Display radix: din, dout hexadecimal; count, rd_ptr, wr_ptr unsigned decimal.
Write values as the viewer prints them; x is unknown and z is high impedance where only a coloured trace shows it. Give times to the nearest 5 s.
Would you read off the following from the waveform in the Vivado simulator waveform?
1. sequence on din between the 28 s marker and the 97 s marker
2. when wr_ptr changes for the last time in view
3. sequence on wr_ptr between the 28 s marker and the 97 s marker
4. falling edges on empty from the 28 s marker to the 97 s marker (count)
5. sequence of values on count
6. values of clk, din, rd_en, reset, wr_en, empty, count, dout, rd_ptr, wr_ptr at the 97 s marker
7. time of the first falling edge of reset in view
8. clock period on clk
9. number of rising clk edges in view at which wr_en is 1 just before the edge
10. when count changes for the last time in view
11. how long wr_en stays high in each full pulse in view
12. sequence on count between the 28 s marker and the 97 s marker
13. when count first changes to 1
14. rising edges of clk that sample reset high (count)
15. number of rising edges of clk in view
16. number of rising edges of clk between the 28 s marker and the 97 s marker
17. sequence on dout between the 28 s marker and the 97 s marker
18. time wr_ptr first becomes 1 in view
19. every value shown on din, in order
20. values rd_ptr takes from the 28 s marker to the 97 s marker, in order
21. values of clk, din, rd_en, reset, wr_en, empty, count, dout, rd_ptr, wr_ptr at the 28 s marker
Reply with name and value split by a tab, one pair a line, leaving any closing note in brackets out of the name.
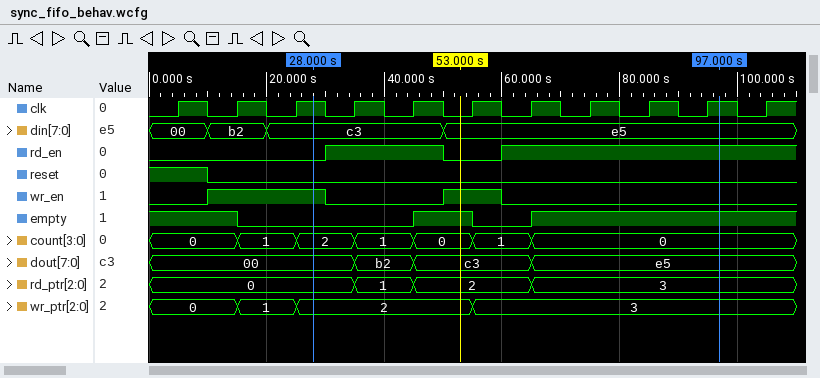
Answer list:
sequence on din between the 28 s marker and the 97 s marker	c3, e5
when wr_ptr changes for the last time in view	55 s
sequence on wr_ptr between the 28 s marker and the 97 s marker	2, 3
falling edges on empty from the 28 s marker to the 97 s marker	1
sequence of values on count	0, 1, 2, 1, 0, 1, 0
values of clk, din, rd_en, reset, wr_en, empty, count, dout, rd_ptr, wr_ptr at the 97 s marker	clk=1, din=e5, rd_en=1, reset=0, wr_en=0, empty=1, count=0, dout=e5, rd_ptr=3, wr_ptr=3
time of the first falling edge of reset in view	10 s
clock period on clk	10 s
number of rising clk edges in view at which wr_en is 1 just before the edge	3
when count changes for the last time in view	65 s
how long wr_en stays high in each full pulse in view	20 s, 10 s
sequence on count between the 28 s marker and the 97 s marker	2, 1, 0, 1, 0
when count first changes to 1	15 s
rising edges of clk that sample reset high	1
number of rising edges of clk in view	11
number of rising edges of clk between the 28 s marker and the 97 s marker	7
sequence on dout between the 28 s marker and the 97 s marker	00, b2, c3, e5
time wr_ptr first becomes 1 in view	15 s
every value shown on din, in order	00, b2, c3, e5
values rd_ptr takes from the 28 s marker to the 97 s marker, in order	0, 1, 2, 3
values of clk, din, rd_en, reset, wr_en, empty, count, dout, rd_ptr, wr_ptr at the 28 s marker	clk=1, din=c3, rd_en=0, reset=0, wr_en=1, empty=0, count=2, dout=00, rd_ptr=0, wr_ptr=2
